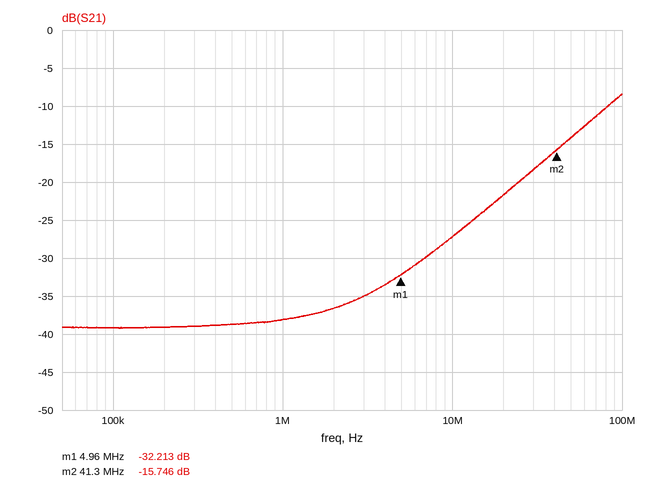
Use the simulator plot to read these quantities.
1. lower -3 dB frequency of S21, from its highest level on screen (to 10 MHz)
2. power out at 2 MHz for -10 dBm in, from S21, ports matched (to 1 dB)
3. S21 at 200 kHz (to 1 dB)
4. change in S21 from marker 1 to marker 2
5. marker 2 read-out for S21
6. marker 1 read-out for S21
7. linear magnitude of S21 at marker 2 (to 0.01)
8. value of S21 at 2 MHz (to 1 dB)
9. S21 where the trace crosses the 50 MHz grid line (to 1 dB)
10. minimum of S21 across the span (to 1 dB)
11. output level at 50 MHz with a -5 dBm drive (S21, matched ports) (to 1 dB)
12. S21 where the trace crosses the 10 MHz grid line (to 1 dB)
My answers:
70 MHz
-47 dBm
-39 dB
16.467 dB
-15.746 dB
-32.213 dB
0.16
-37 dB
-14 dB
-39 dB
-19 dBm
-27 dB
